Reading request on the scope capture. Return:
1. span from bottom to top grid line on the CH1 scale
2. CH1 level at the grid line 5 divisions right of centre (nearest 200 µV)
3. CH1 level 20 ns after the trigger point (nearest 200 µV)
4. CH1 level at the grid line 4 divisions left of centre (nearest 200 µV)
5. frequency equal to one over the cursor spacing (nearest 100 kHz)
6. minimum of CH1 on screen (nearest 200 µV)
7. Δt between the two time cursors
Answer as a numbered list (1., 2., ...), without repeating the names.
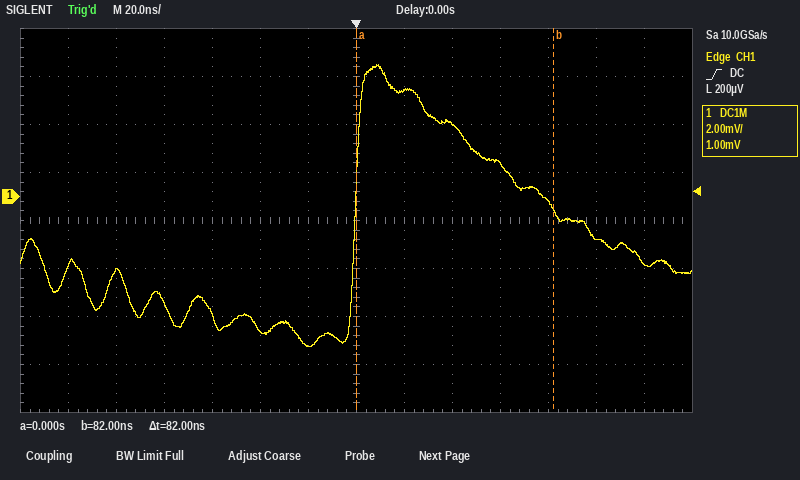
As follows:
1. 16 mV
2. -1.8 mV
3. 4.4 mV
4. -4.4 mV
5. 12.2 MHz
6. -6.2 mV
7. 82 ns
